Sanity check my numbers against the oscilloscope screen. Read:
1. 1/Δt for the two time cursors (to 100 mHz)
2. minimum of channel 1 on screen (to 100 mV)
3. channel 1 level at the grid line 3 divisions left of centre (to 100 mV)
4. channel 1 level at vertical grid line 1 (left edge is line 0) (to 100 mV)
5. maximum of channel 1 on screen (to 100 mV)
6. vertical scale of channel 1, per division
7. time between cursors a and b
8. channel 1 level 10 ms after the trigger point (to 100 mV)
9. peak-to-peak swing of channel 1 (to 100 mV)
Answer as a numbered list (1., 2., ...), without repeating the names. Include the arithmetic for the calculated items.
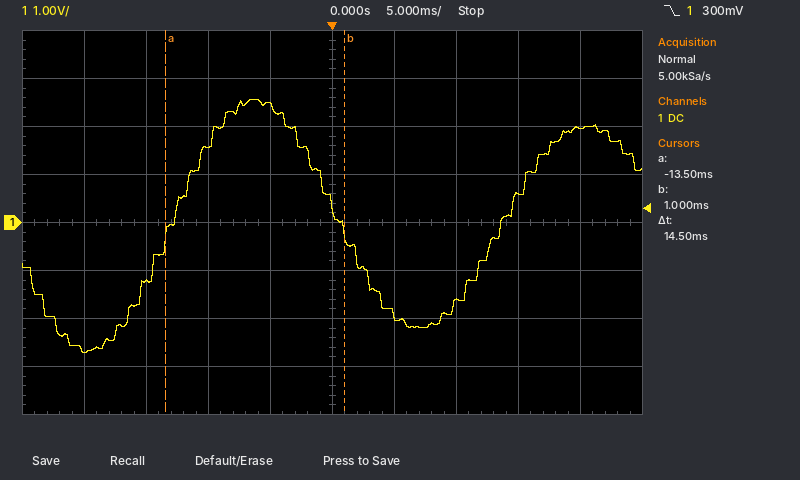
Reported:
1. 1 / 14.5 ms ≈ 69.0 Hz
2. -2.7 V
3. -1.2 V
4. -2.7 V
5. 2.6 V
6. 1 V
7. 14.5 ms
8. -1.7 V
9. 2.6 V − (-2.7 V) = 5.3 V
